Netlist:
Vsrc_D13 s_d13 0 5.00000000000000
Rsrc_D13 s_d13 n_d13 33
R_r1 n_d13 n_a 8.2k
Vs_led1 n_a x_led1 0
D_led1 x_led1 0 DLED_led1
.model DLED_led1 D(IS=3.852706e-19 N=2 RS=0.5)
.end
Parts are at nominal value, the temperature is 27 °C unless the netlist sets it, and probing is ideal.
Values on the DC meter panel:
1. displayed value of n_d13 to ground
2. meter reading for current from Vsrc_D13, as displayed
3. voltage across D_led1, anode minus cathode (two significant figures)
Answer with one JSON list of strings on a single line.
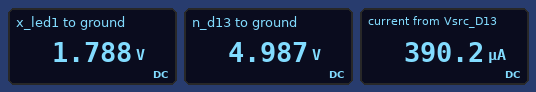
["4.987 V", "390.2 µA", "1.8 V"]
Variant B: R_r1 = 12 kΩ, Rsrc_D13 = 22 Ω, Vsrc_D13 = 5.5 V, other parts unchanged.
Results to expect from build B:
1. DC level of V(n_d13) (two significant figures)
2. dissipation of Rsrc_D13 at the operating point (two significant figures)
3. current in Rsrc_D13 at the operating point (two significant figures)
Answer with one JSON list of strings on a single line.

["5.5 V", "2.1 µW", "310 µA"]
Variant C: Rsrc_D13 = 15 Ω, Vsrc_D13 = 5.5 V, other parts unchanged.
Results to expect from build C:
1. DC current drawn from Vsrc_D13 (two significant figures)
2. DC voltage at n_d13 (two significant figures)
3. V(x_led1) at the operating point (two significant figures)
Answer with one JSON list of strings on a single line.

["450 µA", "5.5 V", "1.8 V"]
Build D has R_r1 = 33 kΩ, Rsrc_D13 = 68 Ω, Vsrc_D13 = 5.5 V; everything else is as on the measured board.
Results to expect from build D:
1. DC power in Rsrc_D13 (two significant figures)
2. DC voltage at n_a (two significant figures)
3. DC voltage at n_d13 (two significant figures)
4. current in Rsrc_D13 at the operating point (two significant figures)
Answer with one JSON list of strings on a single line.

["890 nW", "1.7 V", "5.5 V", "110 µA"]
